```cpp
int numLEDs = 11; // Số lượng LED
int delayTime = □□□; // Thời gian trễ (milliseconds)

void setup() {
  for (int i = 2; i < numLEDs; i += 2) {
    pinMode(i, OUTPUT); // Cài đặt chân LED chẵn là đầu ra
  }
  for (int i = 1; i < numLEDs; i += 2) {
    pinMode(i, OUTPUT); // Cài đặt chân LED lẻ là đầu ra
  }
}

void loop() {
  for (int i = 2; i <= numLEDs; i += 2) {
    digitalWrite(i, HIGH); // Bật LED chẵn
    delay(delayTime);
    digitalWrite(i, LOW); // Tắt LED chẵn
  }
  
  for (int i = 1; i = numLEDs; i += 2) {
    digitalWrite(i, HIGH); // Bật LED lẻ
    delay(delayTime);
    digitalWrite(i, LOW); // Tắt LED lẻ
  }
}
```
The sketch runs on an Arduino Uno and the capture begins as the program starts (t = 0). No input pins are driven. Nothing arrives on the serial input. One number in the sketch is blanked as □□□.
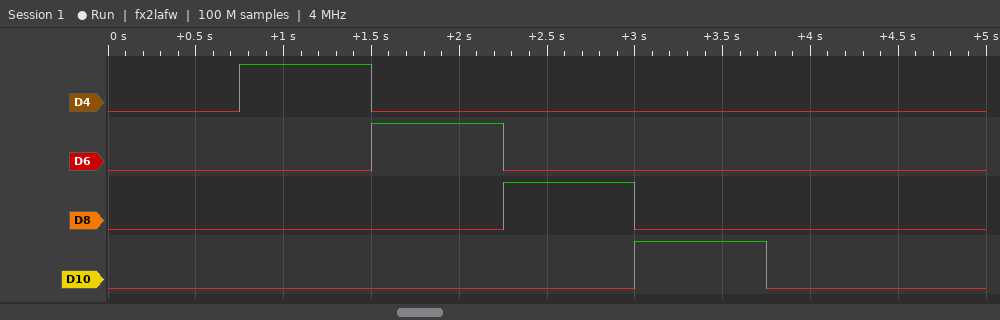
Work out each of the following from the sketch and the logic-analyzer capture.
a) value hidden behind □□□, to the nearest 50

750
